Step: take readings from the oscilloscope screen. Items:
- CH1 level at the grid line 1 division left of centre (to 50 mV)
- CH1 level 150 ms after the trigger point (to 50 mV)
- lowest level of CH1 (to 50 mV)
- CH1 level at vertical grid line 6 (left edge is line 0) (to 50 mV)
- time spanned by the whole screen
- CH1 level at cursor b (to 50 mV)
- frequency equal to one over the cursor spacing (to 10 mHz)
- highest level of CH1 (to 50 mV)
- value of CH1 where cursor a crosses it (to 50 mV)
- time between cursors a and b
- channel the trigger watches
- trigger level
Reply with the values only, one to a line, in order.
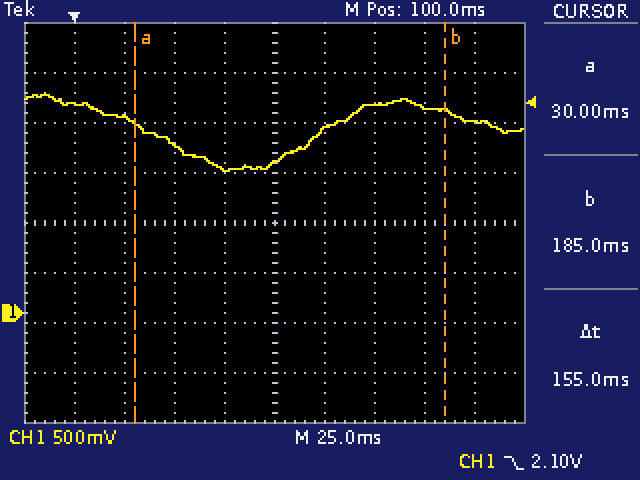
1.45 V
2.10 V
1.40 V
1.85 V
250 ms
2.00 V
6.45 Hz
2.20 V
1.90 V
155 ms
CH1
2.10 V
